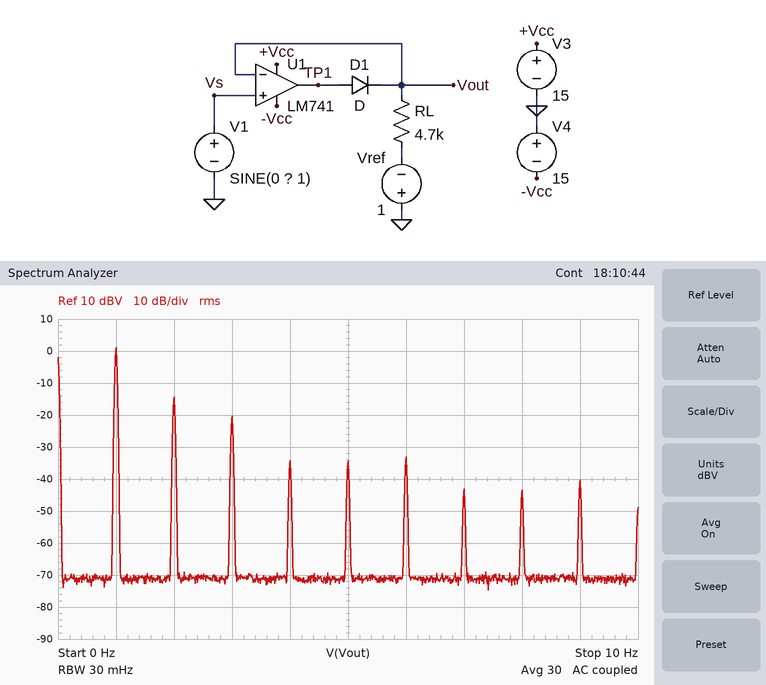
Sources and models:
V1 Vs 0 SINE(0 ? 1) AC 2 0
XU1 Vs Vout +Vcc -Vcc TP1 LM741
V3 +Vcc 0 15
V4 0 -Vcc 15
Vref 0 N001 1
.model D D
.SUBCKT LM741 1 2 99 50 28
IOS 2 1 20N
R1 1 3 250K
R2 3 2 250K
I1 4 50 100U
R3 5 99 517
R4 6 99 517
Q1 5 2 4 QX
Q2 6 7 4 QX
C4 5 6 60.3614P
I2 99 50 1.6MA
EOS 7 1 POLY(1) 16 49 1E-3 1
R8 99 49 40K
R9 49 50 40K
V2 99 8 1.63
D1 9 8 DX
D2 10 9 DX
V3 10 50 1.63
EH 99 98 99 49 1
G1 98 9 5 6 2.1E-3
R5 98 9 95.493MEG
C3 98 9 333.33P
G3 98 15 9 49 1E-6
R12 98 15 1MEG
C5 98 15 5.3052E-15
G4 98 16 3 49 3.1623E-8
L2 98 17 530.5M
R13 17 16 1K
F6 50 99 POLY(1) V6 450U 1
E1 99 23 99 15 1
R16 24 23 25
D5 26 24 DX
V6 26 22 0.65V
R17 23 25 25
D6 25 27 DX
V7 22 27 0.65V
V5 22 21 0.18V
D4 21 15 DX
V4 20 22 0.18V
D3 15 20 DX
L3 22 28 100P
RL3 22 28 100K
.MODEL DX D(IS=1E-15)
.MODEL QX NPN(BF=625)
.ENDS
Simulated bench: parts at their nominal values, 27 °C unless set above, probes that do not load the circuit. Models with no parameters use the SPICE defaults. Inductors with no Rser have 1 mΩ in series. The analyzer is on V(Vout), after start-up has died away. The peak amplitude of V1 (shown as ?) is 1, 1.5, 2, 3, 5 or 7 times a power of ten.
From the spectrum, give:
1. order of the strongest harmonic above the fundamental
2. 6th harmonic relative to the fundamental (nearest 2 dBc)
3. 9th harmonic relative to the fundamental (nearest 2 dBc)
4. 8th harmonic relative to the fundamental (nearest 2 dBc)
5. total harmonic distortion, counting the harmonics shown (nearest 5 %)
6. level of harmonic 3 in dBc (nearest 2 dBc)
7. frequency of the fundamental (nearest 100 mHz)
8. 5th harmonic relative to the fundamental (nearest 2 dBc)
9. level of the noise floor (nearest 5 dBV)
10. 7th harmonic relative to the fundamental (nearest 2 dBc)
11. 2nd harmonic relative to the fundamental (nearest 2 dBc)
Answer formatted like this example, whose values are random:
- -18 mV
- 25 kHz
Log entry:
- 2
- -34 dBc
- -42 dBc
- -44 dBc
- 20 %
- -22 dBc
- 1.0 Hz
- -36 dBc
- -70 dBV
- -44 dBc
- -16 dBc
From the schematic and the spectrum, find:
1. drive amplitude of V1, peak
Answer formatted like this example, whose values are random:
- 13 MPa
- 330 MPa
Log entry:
- 2 V
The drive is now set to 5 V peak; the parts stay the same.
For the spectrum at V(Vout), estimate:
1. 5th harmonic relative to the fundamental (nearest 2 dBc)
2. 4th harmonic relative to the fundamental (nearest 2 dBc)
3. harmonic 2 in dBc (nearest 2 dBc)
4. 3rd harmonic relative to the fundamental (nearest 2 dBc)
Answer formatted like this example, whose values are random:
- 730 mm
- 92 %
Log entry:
- -30 dBc
- -26 dBc
- -10 dBc
- -24 dBc
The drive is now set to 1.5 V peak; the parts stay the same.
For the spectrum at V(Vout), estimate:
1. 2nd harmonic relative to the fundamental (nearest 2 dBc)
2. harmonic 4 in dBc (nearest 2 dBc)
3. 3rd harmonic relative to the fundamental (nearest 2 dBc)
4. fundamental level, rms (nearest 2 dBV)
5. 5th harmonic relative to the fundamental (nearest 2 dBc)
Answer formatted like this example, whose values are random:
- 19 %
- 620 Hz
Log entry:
- -20 dBc
- -30 dBc
- -24 dBc
- 0 dBV
- -42 dBc
